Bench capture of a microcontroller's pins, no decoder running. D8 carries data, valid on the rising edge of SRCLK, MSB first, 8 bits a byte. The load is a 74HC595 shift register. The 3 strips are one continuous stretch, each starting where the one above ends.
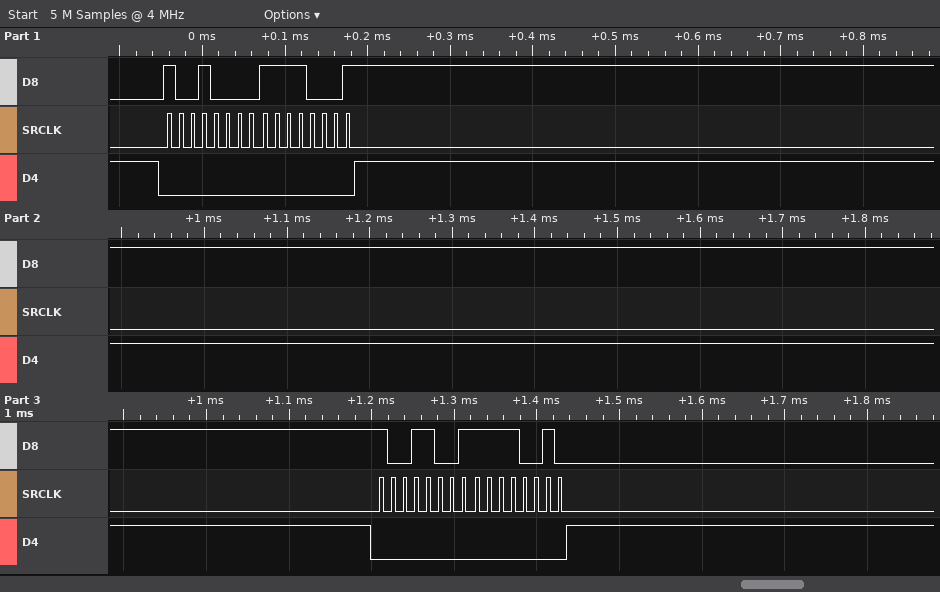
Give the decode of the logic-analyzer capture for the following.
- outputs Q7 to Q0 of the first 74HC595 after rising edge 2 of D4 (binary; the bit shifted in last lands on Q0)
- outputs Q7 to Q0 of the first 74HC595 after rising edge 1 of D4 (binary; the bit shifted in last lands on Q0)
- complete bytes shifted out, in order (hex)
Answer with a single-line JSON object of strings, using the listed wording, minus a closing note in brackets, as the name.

{"outputs Q7 to Q0 of the first 74HC595 after rising edge 2 of D4": "11110010", "outputs Q7 to Q0 of the first 74HC595 after rising edge 1 of D4": "11110001", "complete bytes shifted out, in order": "90 F1 99 F2"}
